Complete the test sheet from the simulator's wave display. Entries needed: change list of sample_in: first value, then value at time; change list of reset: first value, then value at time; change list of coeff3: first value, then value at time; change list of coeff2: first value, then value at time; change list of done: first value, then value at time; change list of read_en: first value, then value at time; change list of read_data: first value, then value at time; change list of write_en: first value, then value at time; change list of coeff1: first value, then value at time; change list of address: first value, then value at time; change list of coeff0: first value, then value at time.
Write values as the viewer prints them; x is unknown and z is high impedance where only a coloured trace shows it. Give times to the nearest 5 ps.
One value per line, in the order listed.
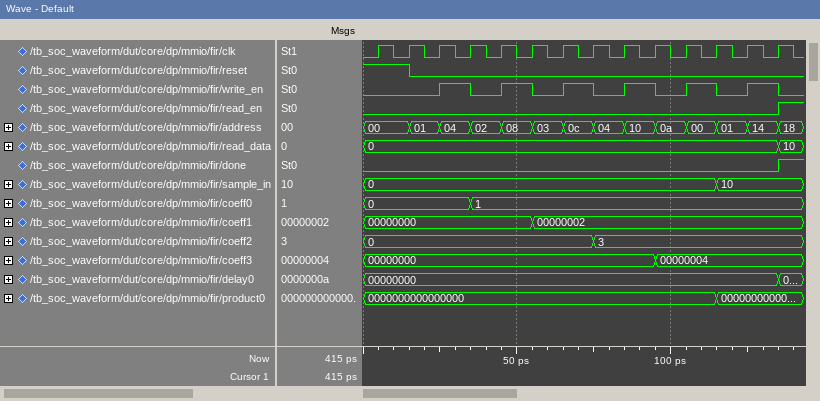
0, 10 at 115 ps
1, 0 at 15 ps
00000000, 00000004 at 95 ps
0, 3 at 75 ps
0, 1 at 135 ps
0, 1 at 135 ps
0, 10 at 135 ps
0, 1 at 25 ps, 0 at 35 ps, 1 at 45 ps, 0 at 55 ps, 1 at 65 ps, 0 at 75 ps, 1 at 85 ps, 0 at 95 ps, 1 at 105 ps, 0 at 115 ps, 1 at 125 ps, 0 at 135 ps
00000000, 00000002 at 55 ps
00, 01 at 15 ps, 04 at 25 ps, 02 at 35 ps, 08 at 45 ps, 03 at 55 ps, 0c at 65 ps, 04 at 75 ps, 10 at 85 ps, 0a at 95 ps, 00 at 105 ps, 01 at 115 ps, 14 at 125 ps, 18 at 135 ps
0, 1 at 35 ps
